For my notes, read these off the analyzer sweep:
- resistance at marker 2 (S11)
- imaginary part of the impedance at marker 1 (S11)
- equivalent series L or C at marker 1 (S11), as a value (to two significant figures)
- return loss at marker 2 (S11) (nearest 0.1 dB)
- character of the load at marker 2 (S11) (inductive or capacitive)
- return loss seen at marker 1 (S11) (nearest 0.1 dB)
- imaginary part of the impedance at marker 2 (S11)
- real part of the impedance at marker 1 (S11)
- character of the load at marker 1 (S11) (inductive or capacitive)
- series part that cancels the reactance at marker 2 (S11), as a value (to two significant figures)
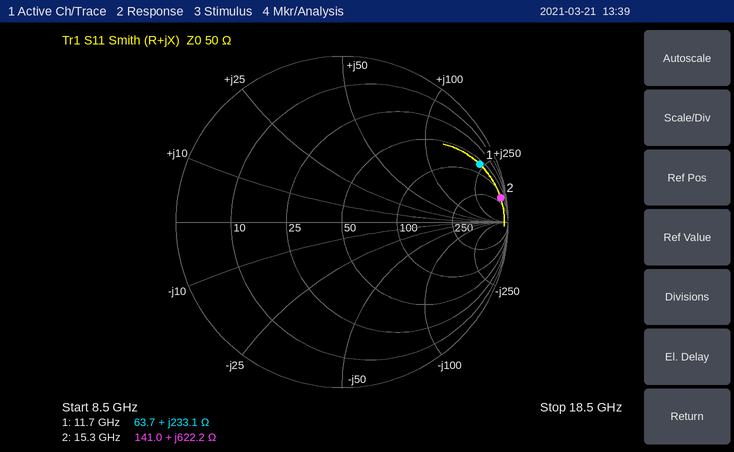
141.0 Ω
+233.1 Ω
3.2 nH
0.3 dB
inductive
0.9 dB
+622.2 Ω
63.7 Ω
inductive
17 fF
